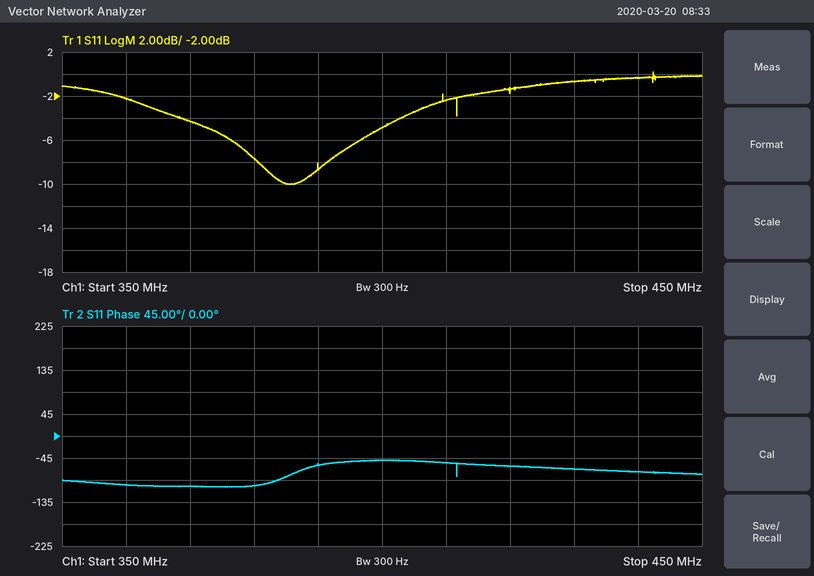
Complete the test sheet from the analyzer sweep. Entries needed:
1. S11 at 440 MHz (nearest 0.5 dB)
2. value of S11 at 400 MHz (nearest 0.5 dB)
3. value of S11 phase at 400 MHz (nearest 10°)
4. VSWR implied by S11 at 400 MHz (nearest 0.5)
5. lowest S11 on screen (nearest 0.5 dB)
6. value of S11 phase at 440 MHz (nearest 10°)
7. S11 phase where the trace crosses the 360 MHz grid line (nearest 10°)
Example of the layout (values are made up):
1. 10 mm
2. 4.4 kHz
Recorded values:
1. -0.5 dB
2. -5.0 dB
3. -50°
4. 3.5
5. -10.0 dB
6. -70°
7. -100°
